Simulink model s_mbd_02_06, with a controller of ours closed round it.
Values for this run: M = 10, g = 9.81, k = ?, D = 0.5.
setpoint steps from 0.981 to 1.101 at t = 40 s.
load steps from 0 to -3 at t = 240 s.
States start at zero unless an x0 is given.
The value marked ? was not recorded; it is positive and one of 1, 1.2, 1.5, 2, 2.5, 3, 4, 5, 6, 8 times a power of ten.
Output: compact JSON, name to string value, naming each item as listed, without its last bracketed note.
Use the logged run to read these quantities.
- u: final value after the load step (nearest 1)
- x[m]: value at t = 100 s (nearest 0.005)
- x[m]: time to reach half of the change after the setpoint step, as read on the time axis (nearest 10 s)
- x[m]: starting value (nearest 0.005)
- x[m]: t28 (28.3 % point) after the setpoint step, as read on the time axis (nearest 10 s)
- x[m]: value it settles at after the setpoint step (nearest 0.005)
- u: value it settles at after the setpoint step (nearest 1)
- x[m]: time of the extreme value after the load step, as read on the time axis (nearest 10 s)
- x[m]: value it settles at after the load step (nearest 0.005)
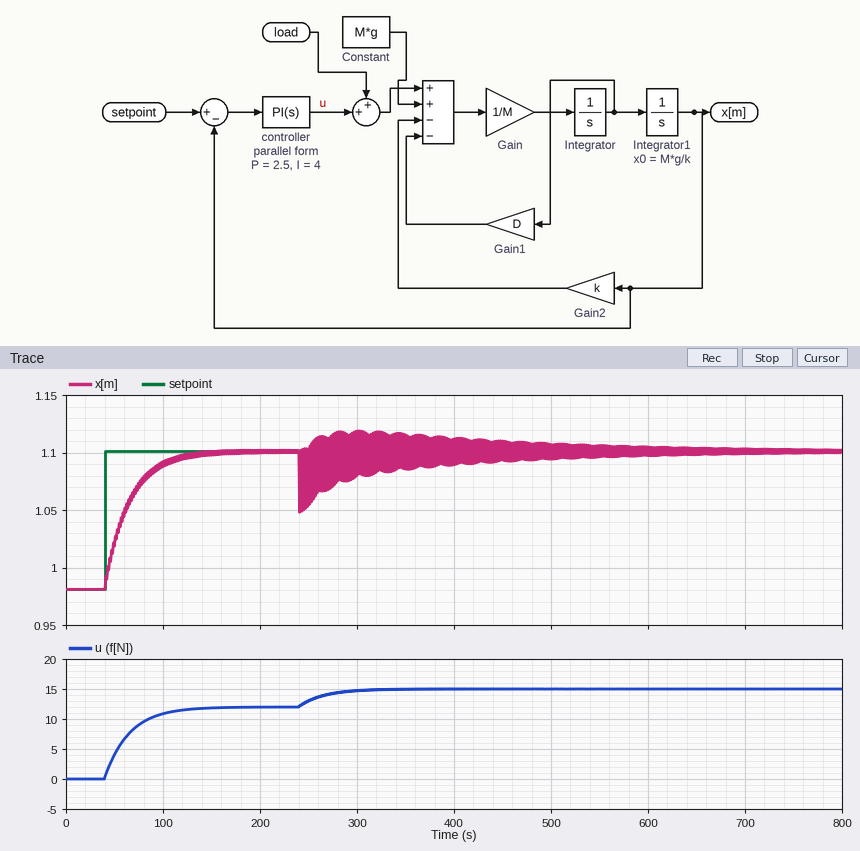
{"u: final value after the load step": "15", "x[m]: value at t = 100 s": "1.090", "x[m]: time to reach half of the change after the setpoint step, as read on the time axis": "60 s", "x[m]: starting value": "0.980", "x[m]: t28 (28.3 % point) after the setpoint step, as read on the time axis": "50 s", "x[m]: value it settles at after the setpoint step": "1.100", "u: value it settles at after the setpoint step": "12", "x[m]: time of the extreme value after the load step, as read on the time axis": "240 s", "x[m]: value it settles at after the load step": "1.100"}
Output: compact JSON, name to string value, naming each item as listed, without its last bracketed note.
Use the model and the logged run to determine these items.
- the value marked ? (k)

{"the value marked ?": "100"}
